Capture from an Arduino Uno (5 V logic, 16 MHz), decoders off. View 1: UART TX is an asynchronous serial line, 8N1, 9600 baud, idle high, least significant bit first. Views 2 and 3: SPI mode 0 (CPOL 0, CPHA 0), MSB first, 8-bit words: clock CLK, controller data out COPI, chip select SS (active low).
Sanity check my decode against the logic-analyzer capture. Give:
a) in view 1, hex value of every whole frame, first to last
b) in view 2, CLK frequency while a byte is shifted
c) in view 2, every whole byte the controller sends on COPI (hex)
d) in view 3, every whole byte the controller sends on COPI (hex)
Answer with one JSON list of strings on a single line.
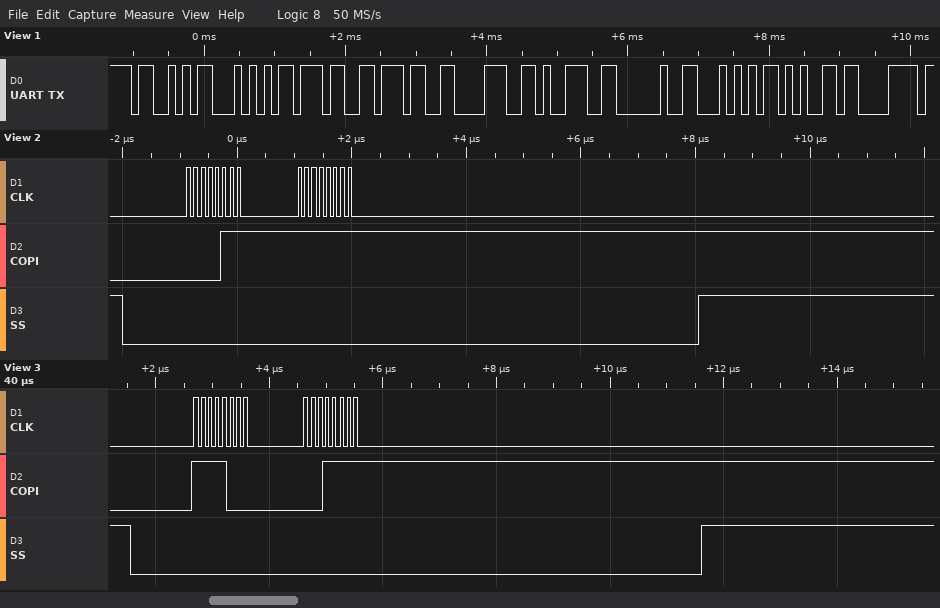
["53 54 37 37 38 39 20 54 65 78", "8 MHz", "0x07 0xFF", "F8 1F"]
